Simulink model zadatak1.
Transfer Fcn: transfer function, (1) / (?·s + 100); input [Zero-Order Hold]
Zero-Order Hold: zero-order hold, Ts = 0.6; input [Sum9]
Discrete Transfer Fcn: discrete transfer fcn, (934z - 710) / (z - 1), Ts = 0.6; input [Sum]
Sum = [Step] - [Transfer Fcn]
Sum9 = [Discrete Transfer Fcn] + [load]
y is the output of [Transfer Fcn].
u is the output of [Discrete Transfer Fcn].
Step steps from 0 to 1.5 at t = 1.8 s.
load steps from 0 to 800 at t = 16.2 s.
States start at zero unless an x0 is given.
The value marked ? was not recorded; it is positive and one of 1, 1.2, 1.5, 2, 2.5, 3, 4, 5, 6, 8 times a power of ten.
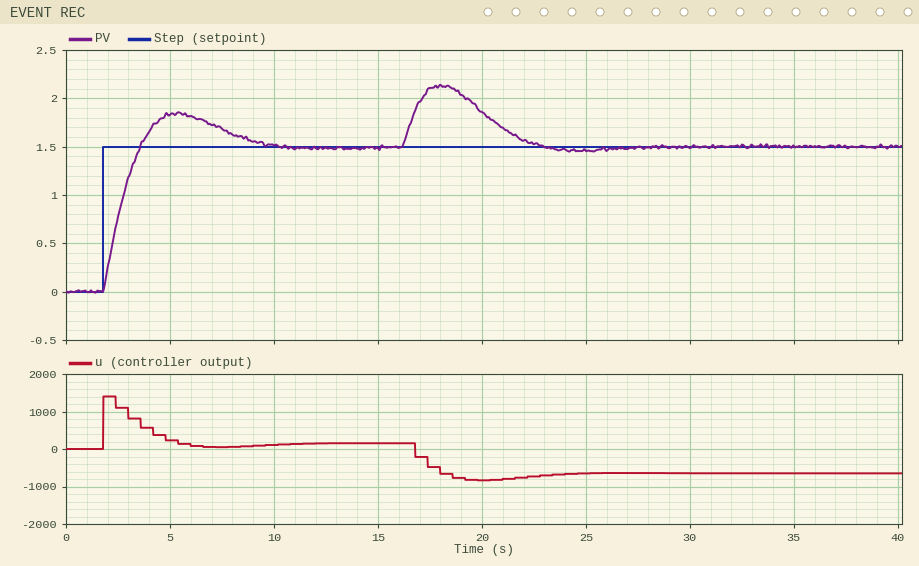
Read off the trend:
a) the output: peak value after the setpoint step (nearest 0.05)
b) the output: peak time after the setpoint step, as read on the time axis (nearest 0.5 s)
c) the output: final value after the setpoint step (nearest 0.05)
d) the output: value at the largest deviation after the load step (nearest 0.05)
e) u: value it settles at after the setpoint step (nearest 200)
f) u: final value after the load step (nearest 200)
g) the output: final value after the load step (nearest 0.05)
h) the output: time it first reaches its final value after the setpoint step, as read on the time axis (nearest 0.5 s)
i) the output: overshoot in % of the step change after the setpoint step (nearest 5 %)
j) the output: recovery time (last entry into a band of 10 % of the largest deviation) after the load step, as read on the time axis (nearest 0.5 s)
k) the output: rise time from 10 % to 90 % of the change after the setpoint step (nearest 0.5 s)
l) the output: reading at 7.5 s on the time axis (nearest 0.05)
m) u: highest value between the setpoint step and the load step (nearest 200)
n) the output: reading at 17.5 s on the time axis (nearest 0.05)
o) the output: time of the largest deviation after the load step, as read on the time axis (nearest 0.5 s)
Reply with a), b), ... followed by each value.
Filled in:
a) 1.85
b) 5.5 s
c) 1.50
d) 2.15
e) 200
f) -600
g) 1.50
h) 3.5 s
i) 25 %
j) 22.0 s
k) 1.5 s
l) 1.70
m) 1400
n) 2.10
o) 18.0 s
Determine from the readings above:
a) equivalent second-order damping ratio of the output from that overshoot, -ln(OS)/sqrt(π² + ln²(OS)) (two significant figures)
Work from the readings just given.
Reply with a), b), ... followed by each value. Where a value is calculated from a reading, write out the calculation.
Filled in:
a) ln(0.25) = -1.386; 1.386 / sqrt(9.870 + 1.922) = 0.40
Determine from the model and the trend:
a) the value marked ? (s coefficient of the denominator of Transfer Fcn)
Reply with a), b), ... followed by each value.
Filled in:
a) 1200
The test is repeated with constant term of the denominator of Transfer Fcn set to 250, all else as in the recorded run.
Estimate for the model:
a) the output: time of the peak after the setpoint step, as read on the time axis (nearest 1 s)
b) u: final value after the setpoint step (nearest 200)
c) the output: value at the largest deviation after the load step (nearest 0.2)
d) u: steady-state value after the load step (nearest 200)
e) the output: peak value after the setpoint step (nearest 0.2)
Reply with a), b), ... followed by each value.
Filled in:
a) 5 s
b) 400
c) 2.0
d) -400
e) 1.6
